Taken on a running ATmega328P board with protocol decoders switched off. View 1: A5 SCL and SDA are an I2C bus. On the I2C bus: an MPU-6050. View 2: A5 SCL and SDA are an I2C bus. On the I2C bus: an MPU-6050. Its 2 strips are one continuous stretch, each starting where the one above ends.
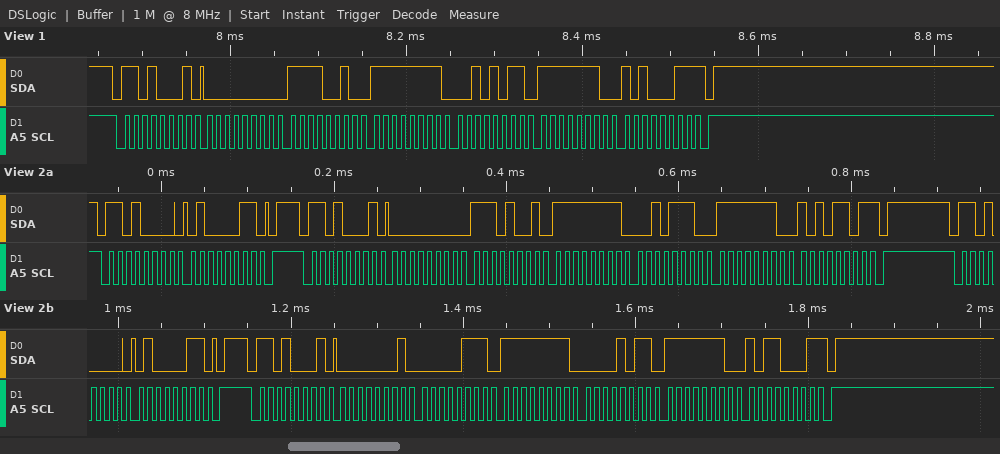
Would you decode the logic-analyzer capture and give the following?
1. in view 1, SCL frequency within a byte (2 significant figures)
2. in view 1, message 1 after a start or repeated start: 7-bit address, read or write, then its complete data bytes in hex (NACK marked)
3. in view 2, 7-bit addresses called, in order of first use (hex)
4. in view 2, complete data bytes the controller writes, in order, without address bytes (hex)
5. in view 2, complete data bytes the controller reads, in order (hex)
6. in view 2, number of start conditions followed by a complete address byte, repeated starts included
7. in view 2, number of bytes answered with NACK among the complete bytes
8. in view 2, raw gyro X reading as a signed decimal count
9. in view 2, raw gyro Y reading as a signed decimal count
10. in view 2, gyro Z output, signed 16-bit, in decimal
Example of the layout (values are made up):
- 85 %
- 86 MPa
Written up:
- 100 kHz
- 0x68 read: 00 F2 FF 2B FE A3 NACK
- 0x68
- 43 43
- 00 E9 FF 2E FE AD 01 07 FF 0B FE B1
- 4
- 2
- 233
- -210
- -339
